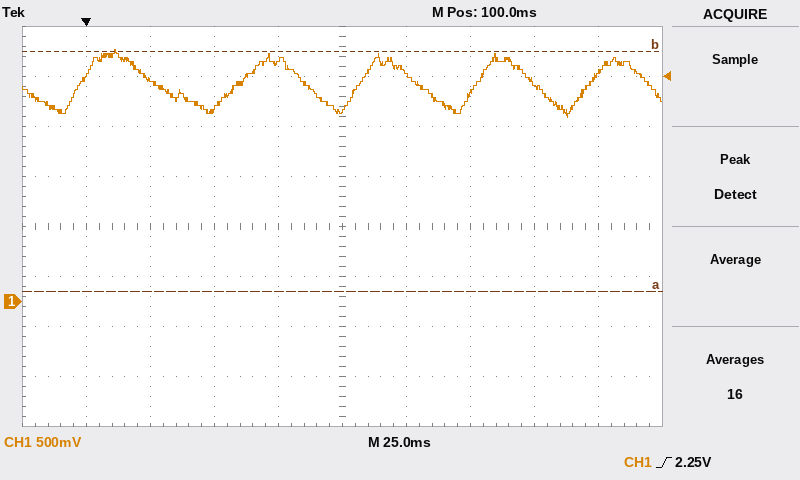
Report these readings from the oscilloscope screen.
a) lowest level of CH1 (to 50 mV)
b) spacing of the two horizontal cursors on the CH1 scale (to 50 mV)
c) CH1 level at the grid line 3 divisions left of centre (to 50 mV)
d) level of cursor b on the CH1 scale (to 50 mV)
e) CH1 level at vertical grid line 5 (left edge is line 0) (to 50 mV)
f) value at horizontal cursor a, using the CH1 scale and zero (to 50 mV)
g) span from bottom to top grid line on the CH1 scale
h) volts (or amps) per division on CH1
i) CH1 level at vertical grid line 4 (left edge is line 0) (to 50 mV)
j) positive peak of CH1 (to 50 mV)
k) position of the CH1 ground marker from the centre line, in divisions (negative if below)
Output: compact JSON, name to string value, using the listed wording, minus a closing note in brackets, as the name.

{"lowest level of CH1": "1.85 V", "spacing of the two horizontal cursors on the CH1 scale": "2.40 V", "CH1 level at the grid line 3 divisions left of centre": "2.20 V", "level of cursor b on the CH1 scale": "2.50 V", "CH1 level at vertical grid line 5 (left edge is line 0)": "1.90 V", "value at horizontal cursor a, using the CH1 scale and zero": "100 mV", "span from bottom to top grid line on the CH1 scale": "4 V", "volts (or amps) per division on CH1": "500 mV", "CH1 level at vertical grid line 4 (left edge is line 0)": "2.40 V", "positive peak of CH1": "2.50 V", "position of the CH1 ground marker from the centre line, in divisions": "-1.5 div"}
